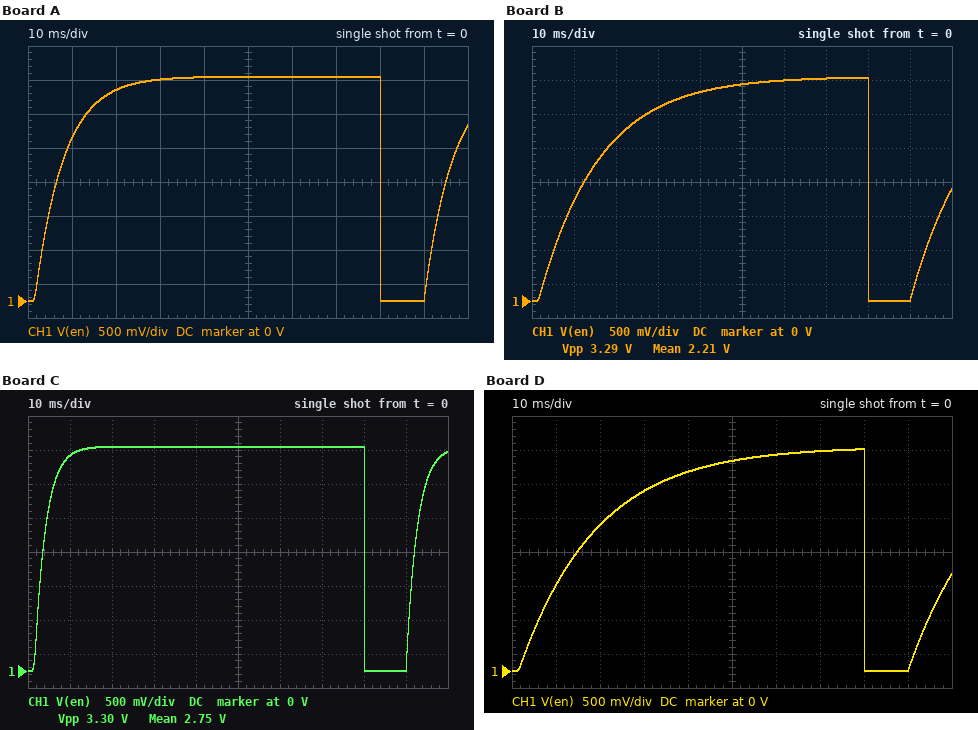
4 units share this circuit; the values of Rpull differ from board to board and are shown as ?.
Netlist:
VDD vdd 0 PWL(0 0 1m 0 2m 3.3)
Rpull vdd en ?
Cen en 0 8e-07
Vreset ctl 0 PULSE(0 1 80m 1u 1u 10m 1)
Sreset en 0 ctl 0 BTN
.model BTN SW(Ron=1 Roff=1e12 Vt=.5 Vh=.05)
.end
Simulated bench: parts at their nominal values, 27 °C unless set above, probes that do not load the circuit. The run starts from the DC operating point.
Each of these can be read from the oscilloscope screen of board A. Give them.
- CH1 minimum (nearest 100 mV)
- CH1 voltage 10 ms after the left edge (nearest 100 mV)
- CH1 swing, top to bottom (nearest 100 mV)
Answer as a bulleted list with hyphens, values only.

- 0 V
- 2.4 V
- 3.3 V
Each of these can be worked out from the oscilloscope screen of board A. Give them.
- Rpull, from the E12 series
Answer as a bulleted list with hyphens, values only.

- 8.2 kΩ
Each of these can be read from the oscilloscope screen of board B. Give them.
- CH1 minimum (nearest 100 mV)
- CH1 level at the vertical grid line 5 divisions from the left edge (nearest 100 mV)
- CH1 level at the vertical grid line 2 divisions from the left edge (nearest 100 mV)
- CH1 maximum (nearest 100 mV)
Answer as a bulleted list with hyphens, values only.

- 0 V
- 3.2 V
- 2.4 V
- 3.3 V
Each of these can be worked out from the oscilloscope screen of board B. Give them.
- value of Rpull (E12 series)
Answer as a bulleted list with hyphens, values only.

- 18 kΩ
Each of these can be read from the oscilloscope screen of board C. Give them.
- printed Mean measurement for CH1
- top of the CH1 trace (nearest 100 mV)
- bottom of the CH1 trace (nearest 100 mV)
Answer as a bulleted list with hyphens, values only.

- 2.75 V
- 3.3 V
- 0 V
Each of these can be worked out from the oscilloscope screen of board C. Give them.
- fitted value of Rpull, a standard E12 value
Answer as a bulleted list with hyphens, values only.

- 3.3 kΩ
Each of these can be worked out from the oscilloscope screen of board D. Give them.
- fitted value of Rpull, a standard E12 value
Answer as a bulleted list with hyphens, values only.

- 22 kΩ
